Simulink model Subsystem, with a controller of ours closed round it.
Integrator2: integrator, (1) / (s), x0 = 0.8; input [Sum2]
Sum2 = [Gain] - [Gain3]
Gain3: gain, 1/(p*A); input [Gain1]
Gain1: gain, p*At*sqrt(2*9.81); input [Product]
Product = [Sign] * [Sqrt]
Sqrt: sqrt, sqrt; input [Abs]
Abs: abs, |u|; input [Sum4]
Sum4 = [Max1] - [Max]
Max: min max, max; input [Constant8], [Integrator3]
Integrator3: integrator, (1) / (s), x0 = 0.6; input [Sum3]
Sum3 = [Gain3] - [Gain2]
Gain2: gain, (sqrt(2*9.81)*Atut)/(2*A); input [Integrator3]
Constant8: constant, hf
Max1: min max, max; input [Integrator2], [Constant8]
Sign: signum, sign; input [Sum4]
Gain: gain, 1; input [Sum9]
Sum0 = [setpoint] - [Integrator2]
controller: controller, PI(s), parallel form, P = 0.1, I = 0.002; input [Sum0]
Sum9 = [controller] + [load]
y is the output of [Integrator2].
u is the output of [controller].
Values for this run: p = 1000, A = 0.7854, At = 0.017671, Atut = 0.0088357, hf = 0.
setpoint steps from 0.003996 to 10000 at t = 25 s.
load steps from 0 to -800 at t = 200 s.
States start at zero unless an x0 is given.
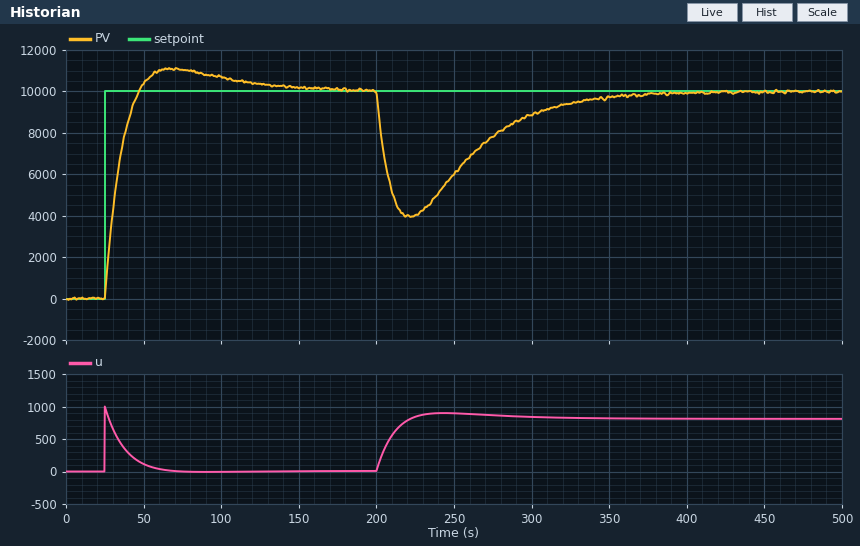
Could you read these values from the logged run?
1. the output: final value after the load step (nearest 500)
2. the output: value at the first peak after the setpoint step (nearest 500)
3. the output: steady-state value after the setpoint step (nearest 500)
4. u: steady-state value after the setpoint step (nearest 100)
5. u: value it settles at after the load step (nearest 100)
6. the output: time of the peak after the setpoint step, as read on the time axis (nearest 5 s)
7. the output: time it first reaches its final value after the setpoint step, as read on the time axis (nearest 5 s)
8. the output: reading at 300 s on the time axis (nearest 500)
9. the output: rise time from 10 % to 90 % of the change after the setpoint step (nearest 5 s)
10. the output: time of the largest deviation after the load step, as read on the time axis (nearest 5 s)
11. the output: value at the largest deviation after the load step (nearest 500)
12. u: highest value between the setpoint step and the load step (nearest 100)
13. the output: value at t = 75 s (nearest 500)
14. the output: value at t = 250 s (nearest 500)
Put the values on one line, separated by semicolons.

10000; 11000; 10000; 0; 800; 70 s; 45 s; 9000; 15 s; 220 s; 4000; 1000; 11000; 6000
